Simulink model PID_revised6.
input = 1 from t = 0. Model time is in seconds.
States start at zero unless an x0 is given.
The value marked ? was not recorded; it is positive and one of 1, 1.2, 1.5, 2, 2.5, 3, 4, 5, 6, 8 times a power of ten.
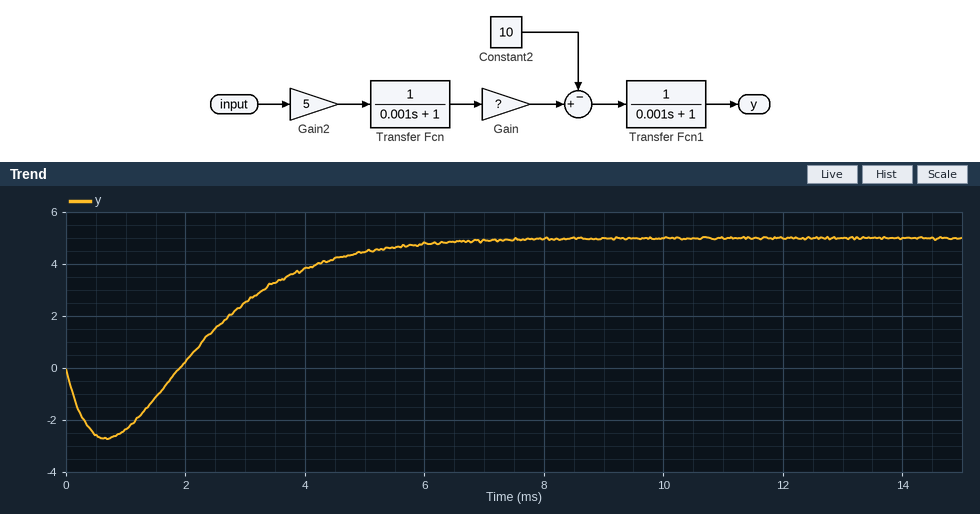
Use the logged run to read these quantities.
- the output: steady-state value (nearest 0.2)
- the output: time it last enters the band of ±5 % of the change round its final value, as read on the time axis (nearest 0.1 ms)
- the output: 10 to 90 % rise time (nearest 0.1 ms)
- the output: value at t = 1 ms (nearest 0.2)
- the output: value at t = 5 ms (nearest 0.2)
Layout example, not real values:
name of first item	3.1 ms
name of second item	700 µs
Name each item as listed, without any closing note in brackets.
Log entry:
the output: steady-state value	5.0
the output: time it last enters the band of ±5 % of the change round its final value, as read on the time axis	5.9 ms
the output: 10 to 90 % rise time	3.0 ms
the output: value at t = 1 ms	-2.4
the output: value at t = 5 ms	4.4
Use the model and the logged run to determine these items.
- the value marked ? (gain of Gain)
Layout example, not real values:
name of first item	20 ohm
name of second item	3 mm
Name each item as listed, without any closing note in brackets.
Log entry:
the value marked ?	3
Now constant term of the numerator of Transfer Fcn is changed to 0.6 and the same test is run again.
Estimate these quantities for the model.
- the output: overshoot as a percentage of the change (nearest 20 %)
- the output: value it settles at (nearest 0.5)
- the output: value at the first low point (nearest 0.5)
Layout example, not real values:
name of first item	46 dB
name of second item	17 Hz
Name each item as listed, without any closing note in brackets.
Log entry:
the output: overshoot as a percentage of the change	300 %
the output: value it settles at	-1.0
the output: value at the first low point	-4.0
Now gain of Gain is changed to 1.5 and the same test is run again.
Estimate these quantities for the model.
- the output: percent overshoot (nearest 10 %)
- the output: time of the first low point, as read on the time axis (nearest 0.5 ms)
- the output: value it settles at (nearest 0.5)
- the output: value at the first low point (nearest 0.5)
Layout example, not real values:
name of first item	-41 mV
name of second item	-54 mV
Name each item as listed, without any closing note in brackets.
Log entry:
the output: percent overshoot	80 %
the output: time of the first low point, as read on the time axis	1.5 ms
the output: value it settles at	-2.5
the output: value at the first low point	-4.5
